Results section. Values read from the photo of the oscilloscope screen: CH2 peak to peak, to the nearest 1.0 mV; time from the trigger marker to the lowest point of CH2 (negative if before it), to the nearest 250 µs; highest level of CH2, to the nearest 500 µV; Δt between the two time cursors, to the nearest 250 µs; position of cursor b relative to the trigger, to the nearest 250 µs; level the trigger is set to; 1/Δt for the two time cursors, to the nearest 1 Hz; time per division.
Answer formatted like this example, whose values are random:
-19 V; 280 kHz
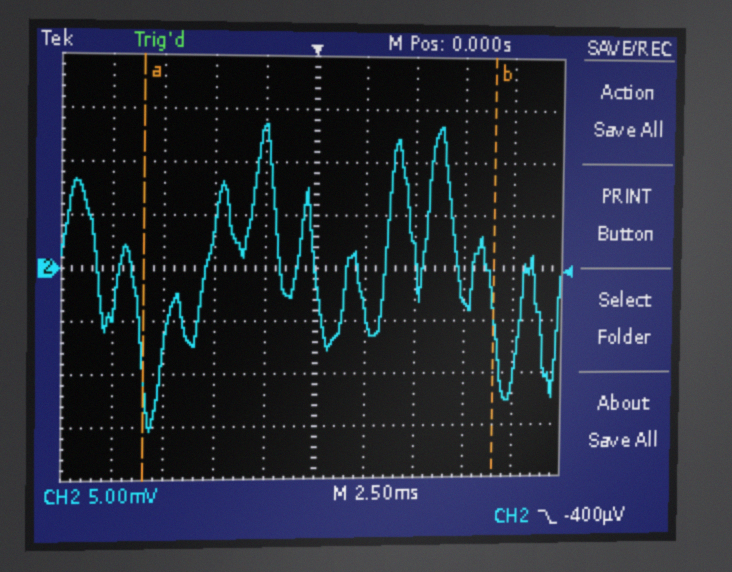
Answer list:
29.0 mV; -8.25 ms; 13.5 mV; 17.50 ms; +9.00 ms; -400 µV; 57 Hz; 2.5 ms
